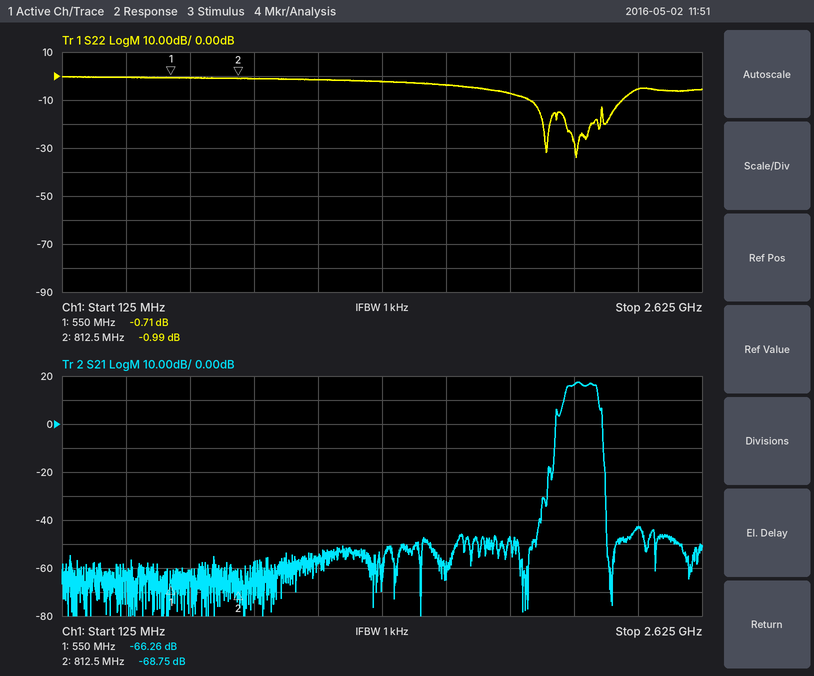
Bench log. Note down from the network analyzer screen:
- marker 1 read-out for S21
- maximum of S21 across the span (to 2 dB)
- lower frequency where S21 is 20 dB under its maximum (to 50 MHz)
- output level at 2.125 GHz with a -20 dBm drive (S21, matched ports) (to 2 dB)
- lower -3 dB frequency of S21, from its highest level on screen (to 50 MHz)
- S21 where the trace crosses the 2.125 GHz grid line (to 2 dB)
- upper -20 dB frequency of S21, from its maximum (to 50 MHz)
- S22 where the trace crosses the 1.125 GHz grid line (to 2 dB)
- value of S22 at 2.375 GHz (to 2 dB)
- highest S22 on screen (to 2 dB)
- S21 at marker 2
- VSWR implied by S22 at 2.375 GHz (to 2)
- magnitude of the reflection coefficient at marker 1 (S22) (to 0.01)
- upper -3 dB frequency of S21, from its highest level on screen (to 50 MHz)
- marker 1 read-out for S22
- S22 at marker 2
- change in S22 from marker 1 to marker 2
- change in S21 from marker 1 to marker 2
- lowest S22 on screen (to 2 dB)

-66.26 dB
18 dB
2.05 GHz
-4 dBm
2.10 GHz
16 dB
2.25 GHz
-2 dB
-6 dB
0 dB
-68.75 dB
4
0.92
2.20 GHz
-0.71 dB
-0.99 dB
-0.28 dB
-2.49 dB
-34 dB
